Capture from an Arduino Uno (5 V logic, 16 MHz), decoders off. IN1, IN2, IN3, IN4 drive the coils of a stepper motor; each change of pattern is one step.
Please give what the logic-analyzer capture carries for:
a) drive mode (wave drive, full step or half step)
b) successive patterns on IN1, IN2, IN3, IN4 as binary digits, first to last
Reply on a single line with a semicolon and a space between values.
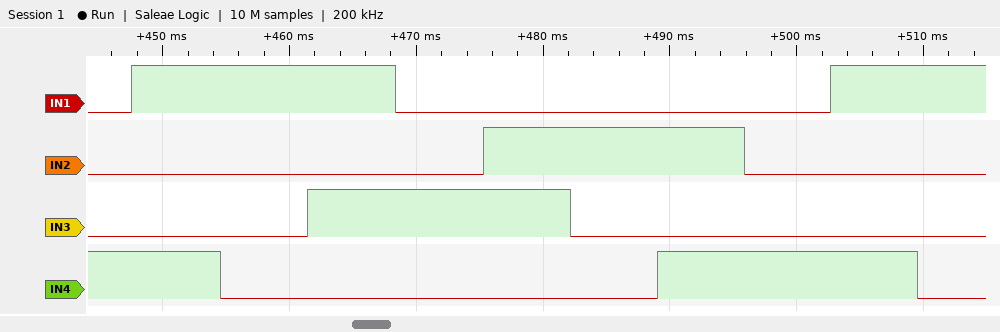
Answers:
half step; 0001 1001 1000 1010 0010 0110 0100 0101 0001 1001 1000
